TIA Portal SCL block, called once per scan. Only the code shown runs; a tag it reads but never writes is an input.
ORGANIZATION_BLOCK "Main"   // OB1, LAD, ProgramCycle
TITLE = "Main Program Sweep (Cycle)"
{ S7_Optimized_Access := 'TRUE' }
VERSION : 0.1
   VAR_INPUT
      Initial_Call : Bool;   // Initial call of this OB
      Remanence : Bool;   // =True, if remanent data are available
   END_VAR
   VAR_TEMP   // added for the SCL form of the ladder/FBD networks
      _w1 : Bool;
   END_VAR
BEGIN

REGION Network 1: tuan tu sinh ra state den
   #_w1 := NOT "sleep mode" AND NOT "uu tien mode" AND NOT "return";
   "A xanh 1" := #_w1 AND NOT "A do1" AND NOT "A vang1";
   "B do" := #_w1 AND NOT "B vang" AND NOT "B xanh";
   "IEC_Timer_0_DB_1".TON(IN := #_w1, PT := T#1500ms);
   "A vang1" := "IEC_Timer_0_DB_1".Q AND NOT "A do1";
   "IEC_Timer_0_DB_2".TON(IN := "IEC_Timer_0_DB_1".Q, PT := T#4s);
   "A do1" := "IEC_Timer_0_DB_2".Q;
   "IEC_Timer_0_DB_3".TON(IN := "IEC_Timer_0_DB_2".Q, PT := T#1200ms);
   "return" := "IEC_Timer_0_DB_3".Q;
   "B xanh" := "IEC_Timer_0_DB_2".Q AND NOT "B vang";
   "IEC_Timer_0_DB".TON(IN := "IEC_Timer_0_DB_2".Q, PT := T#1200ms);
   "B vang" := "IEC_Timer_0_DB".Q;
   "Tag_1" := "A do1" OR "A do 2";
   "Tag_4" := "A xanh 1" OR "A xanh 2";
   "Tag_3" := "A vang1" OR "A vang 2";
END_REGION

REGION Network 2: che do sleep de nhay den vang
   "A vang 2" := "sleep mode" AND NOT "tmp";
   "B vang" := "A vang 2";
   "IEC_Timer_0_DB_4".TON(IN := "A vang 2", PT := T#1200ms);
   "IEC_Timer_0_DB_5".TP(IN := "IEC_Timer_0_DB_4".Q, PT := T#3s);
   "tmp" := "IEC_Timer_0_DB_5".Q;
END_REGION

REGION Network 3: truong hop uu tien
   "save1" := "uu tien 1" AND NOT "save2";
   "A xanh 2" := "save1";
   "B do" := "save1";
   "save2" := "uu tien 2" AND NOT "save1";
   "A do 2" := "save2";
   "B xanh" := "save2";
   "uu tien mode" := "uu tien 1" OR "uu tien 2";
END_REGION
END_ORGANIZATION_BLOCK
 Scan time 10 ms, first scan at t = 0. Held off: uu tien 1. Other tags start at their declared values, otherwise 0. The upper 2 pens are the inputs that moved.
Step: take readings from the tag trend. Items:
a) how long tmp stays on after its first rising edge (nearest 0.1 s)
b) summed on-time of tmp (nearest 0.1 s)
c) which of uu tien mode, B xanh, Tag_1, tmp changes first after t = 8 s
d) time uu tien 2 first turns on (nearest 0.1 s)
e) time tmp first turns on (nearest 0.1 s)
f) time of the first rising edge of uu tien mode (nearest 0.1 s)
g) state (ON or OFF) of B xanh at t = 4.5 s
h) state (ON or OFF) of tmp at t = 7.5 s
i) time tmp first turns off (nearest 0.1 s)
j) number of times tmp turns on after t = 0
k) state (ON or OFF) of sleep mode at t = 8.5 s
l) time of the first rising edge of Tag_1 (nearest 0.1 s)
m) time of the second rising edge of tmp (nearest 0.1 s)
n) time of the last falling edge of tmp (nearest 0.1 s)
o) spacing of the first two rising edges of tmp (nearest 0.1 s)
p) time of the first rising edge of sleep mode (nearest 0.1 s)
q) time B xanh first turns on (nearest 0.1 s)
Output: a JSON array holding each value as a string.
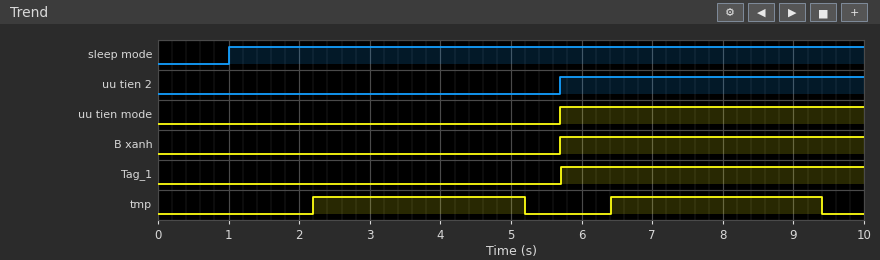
["3.0 s", "6.0 s", "tmp", "5.7 s", "2.2 s", "5.7 s", "OFF", "ON", "5.2 s", "2", "ON", "5.7 s", "6.4 s", "9.4 s", "4.2 s", "1.0 s", "5.7 s"]
